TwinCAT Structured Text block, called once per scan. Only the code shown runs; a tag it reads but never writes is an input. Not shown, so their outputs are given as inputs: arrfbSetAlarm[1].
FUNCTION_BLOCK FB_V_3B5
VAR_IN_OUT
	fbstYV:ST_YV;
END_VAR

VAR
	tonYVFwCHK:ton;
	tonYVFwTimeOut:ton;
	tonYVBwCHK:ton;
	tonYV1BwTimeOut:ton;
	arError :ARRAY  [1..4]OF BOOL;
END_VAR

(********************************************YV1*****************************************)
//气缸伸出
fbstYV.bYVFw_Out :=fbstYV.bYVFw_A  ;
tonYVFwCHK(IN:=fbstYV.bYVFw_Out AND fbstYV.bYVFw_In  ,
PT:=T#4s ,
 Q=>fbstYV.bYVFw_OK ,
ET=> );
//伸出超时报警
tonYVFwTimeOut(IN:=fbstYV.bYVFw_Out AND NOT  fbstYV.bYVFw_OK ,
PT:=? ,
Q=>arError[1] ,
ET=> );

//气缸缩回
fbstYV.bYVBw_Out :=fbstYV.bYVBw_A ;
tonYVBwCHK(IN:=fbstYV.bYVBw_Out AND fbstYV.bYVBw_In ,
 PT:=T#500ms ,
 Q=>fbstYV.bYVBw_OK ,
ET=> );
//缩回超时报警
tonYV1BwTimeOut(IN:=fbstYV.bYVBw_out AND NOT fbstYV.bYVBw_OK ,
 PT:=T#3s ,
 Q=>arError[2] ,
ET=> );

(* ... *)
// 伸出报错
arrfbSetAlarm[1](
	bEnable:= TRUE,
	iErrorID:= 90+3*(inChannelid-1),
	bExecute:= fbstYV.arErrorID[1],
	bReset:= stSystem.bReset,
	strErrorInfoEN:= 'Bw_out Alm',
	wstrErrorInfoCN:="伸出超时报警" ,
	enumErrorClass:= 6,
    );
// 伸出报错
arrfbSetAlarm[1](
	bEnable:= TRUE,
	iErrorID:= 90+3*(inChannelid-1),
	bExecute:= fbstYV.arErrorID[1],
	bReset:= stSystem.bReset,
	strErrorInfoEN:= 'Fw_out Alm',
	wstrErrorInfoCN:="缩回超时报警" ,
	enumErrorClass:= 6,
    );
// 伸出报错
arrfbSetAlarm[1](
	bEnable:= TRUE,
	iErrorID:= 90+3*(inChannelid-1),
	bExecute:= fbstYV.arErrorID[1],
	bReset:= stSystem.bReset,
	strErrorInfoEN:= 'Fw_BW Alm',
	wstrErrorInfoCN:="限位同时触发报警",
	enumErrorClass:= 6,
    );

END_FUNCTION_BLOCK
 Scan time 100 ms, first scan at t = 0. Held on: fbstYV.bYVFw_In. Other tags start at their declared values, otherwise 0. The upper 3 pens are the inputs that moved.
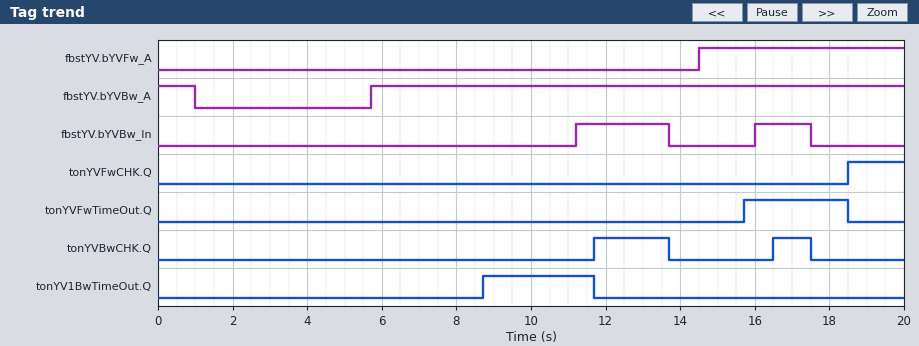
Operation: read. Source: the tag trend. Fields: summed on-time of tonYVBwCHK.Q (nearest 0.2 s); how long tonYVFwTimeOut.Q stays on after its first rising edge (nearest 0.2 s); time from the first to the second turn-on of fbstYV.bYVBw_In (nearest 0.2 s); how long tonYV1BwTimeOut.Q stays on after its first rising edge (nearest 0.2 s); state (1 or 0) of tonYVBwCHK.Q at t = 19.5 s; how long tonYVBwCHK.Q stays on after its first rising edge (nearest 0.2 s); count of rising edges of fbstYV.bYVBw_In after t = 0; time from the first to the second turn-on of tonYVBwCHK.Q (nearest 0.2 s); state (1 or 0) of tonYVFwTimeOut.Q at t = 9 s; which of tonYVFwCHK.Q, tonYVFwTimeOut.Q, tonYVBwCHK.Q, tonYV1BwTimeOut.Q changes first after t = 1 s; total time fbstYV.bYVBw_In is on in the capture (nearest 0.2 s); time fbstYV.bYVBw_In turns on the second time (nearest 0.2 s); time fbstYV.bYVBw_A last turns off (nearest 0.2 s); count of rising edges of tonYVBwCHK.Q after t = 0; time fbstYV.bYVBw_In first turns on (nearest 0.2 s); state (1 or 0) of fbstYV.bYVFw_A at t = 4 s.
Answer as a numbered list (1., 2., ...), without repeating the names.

1. 3.0 s
2. 2.8 s
3. 4.8 s
4. 3.0 s
5. 0
6. 2.0 s
7. 2
8. 4.8 s
9. 0
10. tonYV1BwTimeOut.Q
11. 4.0 s
12. 16.0 s
13. 1.0 s
14. 2
15. 11.2 s
16. 0
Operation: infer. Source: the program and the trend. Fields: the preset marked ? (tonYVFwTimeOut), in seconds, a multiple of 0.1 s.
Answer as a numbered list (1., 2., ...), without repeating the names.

1. 1.2 s
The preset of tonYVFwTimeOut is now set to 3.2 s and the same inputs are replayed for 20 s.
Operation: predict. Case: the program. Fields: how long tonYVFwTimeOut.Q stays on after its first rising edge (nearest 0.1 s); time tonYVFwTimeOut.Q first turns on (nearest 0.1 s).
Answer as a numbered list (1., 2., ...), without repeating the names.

1. 0.8 s
2. 17.7 s
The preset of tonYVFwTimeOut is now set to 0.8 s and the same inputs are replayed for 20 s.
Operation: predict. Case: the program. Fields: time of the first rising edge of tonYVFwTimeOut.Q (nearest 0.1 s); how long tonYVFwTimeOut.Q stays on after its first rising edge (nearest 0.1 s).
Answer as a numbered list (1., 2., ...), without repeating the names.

1. 15.3 s
2. 3.2 s
